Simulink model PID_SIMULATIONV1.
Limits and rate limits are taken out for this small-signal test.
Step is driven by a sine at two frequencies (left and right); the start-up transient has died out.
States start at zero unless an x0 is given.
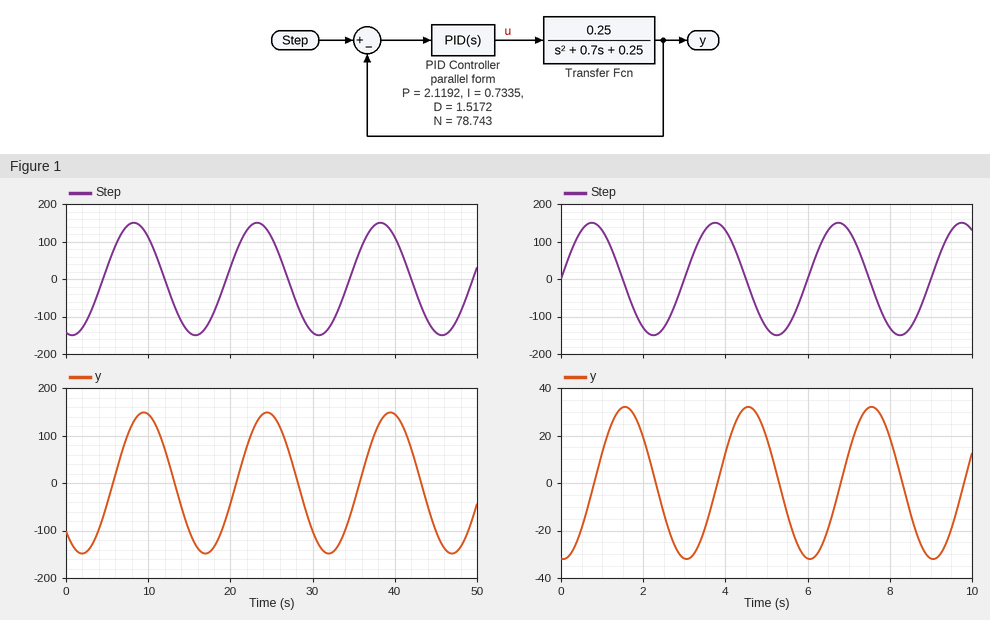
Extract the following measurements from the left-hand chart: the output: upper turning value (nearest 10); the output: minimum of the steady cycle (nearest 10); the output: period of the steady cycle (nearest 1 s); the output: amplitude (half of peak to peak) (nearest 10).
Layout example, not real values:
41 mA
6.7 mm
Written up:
150
-150
15 s
150
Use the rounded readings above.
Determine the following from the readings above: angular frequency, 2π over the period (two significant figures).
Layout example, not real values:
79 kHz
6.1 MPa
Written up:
0.42 rad/s
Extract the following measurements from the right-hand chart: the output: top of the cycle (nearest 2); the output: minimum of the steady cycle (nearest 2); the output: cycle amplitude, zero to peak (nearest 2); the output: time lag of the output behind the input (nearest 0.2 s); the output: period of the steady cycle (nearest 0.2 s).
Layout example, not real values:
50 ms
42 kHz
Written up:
32
-32
32
0.8 s
3.0 s
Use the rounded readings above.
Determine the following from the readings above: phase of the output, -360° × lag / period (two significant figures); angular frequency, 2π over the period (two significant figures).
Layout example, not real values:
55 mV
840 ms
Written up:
-96°
2.1 rad/s
